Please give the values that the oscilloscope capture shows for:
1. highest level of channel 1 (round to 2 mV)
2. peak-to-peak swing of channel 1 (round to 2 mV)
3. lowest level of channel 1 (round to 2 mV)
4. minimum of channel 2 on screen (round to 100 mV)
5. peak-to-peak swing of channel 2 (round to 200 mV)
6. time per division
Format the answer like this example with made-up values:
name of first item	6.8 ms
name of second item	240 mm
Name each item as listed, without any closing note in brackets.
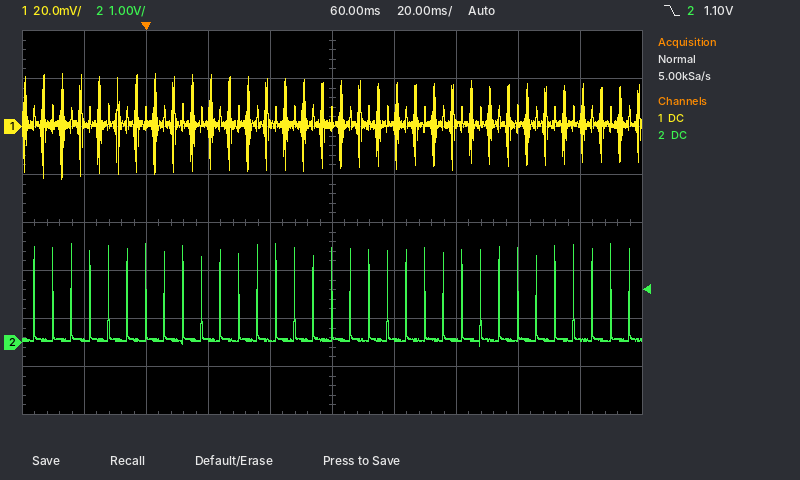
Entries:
highest level of channel 1	22 mV
peak-to-peak swing of channel 1	44 mV
lowest level of channel 1	-22 mV
minimum of channel 2 on screen	-100 mV
peak-to-peak swing of channel 2	2.2 V
time per division	20 ms
